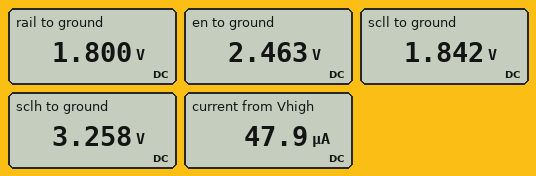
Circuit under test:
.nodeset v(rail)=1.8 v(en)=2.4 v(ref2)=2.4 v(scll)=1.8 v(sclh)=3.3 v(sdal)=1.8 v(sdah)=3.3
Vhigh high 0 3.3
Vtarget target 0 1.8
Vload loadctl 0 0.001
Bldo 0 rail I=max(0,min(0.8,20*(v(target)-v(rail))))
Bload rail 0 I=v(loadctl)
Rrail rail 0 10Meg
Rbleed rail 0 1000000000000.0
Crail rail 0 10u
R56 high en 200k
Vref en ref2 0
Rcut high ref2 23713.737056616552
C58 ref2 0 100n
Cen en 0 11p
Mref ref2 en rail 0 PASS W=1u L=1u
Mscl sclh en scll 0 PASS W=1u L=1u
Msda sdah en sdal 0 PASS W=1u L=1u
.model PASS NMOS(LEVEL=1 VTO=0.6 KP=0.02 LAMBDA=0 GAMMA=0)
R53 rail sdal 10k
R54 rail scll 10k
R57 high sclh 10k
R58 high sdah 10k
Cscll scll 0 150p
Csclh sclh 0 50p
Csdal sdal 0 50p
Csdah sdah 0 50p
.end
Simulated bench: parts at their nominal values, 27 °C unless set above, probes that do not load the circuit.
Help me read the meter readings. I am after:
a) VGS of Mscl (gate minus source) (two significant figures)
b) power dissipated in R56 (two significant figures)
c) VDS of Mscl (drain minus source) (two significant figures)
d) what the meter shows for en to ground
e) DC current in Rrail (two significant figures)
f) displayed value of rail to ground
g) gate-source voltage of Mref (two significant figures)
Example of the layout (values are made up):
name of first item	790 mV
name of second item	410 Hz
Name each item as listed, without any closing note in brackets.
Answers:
VGS of Mscl (gate minus source)	620 mV
power dissipated in R56	3.5 µW
VDS of Mscl (drain minus source)	1.4 V
what the meter shows for en to ground	2.463 V
DC current in Rrail	180 nA
displayed value of rail to ground	1.800 V
gate-source voltage of Mref	660 mV
